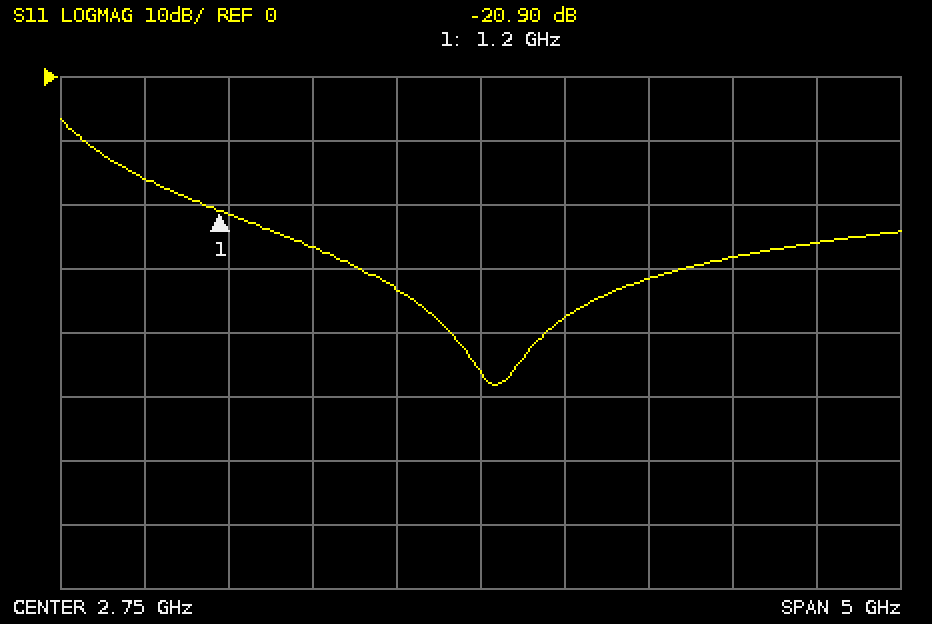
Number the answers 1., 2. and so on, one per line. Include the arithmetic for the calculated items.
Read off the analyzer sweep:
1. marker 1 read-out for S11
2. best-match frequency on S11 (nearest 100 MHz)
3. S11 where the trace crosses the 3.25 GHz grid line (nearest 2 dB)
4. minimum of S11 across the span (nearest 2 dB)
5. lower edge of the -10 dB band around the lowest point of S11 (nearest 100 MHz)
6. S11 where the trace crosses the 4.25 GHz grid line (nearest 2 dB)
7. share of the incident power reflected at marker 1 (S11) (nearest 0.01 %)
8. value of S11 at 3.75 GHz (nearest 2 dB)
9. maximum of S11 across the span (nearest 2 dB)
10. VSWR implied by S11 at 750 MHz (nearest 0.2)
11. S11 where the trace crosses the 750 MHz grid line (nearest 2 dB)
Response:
1. -20.90 dB
2. 2.8 GHz
3. -38 dB
4. -48 dB
5. 400 MHz
6. -28 dB
7. 10^(-20.9/10) ≈ 0.81 %
8. -32 dB
9. -6 dB
10. |Γ| = 10^(-16/20) = 0.1585; VSWR = (1 + 0.1585)/(1 − 0.1585) ≈ 1.4
11. -16 dB
